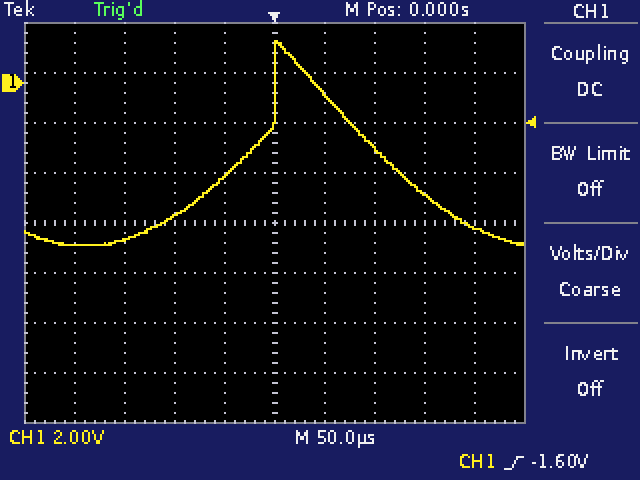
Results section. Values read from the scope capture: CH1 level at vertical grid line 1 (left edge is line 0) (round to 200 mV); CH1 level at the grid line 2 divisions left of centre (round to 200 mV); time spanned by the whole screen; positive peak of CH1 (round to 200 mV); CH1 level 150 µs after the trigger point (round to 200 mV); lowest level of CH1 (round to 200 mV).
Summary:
-6.4 V
-5.4 V
500 µs
1.6 V
-4.4 V
-6.4 V
